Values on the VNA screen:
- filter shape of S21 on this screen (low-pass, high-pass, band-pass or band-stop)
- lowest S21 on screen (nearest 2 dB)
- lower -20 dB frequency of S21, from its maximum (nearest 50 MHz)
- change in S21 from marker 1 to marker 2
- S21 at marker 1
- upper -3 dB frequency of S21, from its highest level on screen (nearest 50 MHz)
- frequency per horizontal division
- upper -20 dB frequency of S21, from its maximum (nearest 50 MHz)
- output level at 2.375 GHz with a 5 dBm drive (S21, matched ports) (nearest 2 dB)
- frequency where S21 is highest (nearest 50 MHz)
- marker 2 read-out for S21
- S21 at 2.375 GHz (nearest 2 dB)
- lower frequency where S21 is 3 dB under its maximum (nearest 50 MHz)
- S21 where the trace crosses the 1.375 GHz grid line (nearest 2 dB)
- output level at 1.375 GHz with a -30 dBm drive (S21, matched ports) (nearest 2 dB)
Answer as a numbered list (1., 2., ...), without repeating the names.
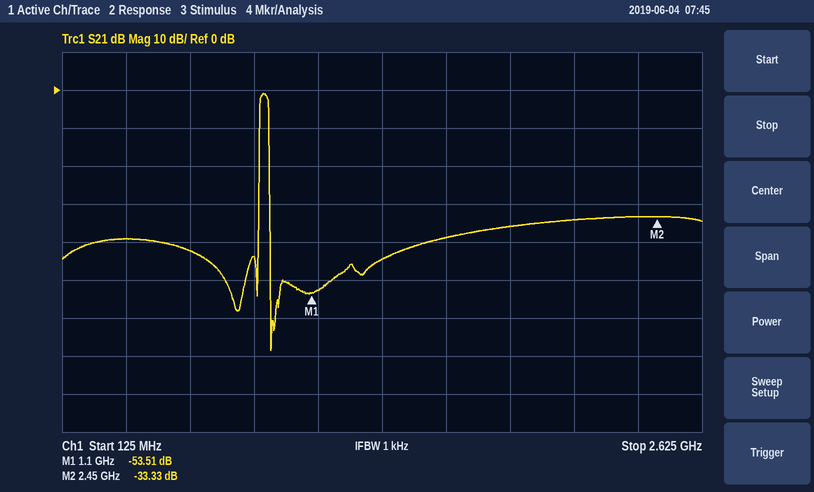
1. band-pass
2. -68 dB
3. 900 MHz
4. 20.18 dB
5. -53.51 dB
6. 950 MHz
7. 250 MHz
8. 950 MHz
9. -28 dBm
10. 900 MHz
11. -33.33 dB
12. -34 dB
13. 900 MHz
14. -44 dB
15. -74 dBm
